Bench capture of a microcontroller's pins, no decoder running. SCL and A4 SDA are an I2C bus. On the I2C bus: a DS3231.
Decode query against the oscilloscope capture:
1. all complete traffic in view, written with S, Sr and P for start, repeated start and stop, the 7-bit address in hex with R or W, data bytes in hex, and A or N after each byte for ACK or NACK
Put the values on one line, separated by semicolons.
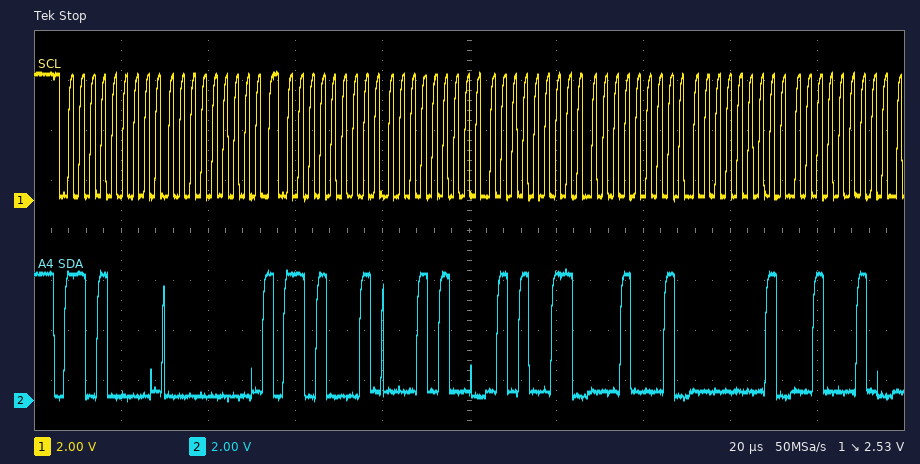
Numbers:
S 68W A 00 A Sr 68R A 14 A 53 A 11 A 01 A 22 A
